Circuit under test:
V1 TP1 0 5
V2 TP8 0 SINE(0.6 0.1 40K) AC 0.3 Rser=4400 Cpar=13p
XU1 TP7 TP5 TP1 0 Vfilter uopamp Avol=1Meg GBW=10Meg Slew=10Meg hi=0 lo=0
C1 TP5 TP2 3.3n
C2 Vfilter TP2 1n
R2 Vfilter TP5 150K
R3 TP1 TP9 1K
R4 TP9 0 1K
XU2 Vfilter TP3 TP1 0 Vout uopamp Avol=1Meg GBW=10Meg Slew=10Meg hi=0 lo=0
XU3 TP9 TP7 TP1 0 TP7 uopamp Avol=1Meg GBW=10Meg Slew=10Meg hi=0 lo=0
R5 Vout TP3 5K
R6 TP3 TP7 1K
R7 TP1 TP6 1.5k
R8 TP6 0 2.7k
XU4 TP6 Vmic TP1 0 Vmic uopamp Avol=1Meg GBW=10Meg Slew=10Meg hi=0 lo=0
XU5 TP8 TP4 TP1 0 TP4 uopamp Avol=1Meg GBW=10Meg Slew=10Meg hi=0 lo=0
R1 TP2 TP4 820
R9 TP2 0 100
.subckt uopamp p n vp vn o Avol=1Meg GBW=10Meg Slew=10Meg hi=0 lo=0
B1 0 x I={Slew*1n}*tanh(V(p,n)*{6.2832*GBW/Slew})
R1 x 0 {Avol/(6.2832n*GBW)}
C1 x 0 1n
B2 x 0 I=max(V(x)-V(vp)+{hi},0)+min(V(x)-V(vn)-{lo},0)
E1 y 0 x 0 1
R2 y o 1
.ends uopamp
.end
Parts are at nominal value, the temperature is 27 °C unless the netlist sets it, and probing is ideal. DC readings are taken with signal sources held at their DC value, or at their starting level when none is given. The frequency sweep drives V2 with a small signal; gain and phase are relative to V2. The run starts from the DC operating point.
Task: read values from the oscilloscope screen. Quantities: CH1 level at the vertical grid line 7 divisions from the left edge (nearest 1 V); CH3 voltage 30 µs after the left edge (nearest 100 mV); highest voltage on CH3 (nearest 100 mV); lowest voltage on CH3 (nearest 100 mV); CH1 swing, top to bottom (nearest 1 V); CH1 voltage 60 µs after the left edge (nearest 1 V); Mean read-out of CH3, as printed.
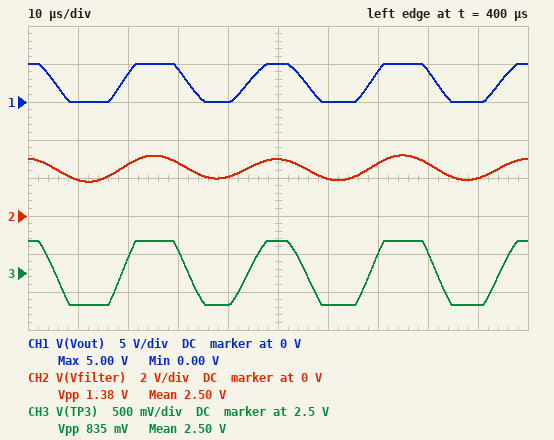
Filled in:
4 V
2.8 V
2.9 V
2.1 V
5 V
0 V
2.50 V
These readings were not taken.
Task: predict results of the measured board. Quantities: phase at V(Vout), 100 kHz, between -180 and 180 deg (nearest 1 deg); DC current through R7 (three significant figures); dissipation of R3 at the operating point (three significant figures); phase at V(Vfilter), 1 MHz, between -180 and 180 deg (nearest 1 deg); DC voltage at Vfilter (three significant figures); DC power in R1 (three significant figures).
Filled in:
84 deg
1.19 mA
6.25 mW
60 deg
2.50 V
349 µW
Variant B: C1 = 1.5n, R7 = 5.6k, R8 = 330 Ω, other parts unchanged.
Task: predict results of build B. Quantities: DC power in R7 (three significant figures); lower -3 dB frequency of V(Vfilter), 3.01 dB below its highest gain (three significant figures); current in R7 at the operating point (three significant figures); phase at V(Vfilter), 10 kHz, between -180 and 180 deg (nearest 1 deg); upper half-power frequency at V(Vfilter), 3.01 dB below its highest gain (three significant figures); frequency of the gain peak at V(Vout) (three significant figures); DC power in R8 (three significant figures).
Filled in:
3.98 mW
32.0 kHz
843 µA
-91 deg
33.5 kHz
32.7 kHz
235 µW
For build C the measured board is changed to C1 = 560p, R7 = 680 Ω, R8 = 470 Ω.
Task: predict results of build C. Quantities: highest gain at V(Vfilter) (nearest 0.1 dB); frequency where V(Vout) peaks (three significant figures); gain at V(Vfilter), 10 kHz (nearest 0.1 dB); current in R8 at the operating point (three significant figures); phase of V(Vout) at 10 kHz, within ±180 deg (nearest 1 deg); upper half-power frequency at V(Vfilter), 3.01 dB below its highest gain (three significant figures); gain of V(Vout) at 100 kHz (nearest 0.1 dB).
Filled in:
36.2 dB
53.6 kHz
-4.5 dB
4.35 mA
-91 deg
54.9 kHz
22.8 dB
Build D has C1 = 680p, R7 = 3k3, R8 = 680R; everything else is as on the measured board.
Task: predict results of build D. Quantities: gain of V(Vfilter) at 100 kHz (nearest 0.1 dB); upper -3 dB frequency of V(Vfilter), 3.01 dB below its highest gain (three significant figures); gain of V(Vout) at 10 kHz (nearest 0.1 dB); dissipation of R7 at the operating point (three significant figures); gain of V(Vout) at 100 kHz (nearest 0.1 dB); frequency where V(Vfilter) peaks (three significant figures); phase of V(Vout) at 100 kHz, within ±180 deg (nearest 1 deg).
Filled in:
6.7 dB
49.8 kHz
12.8 dB
5.21 mW
22.2 dB
48.6 kHz
85 deg
